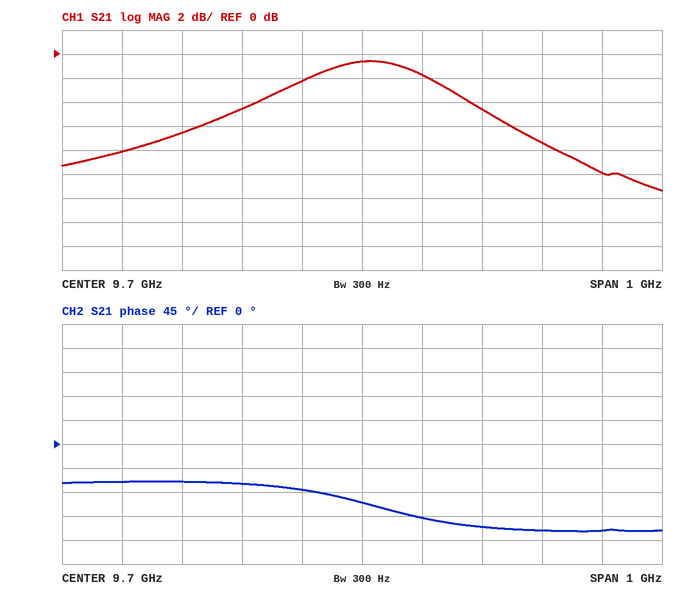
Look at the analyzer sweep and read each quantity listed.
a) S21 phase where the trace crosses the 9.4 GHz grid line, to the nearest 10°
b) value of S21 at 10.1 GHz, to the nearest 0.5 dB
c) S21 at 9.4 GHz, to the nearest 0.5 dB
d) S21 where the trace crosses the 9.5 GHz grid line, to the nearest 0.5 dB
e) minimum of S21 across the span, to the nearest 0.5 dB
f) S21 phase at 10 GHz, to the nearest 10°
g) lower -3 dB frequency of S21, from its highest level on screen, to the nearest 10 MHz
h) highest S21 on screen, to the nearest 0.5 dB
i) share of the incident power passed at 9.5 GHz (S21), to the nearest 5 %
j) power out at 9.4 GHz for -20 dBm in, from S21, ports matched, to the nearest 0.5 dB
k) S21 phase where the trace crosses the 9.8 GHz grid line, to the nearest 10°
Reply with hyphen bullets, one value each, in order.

- -70°
- -10.0 dB
- -6.5 dB
- -4.5 dB
- -11.5 dB
- -160°
- 9.54 GHz
- -0.5 dB
- 35 %
- -26.5 dBm
- -140°
